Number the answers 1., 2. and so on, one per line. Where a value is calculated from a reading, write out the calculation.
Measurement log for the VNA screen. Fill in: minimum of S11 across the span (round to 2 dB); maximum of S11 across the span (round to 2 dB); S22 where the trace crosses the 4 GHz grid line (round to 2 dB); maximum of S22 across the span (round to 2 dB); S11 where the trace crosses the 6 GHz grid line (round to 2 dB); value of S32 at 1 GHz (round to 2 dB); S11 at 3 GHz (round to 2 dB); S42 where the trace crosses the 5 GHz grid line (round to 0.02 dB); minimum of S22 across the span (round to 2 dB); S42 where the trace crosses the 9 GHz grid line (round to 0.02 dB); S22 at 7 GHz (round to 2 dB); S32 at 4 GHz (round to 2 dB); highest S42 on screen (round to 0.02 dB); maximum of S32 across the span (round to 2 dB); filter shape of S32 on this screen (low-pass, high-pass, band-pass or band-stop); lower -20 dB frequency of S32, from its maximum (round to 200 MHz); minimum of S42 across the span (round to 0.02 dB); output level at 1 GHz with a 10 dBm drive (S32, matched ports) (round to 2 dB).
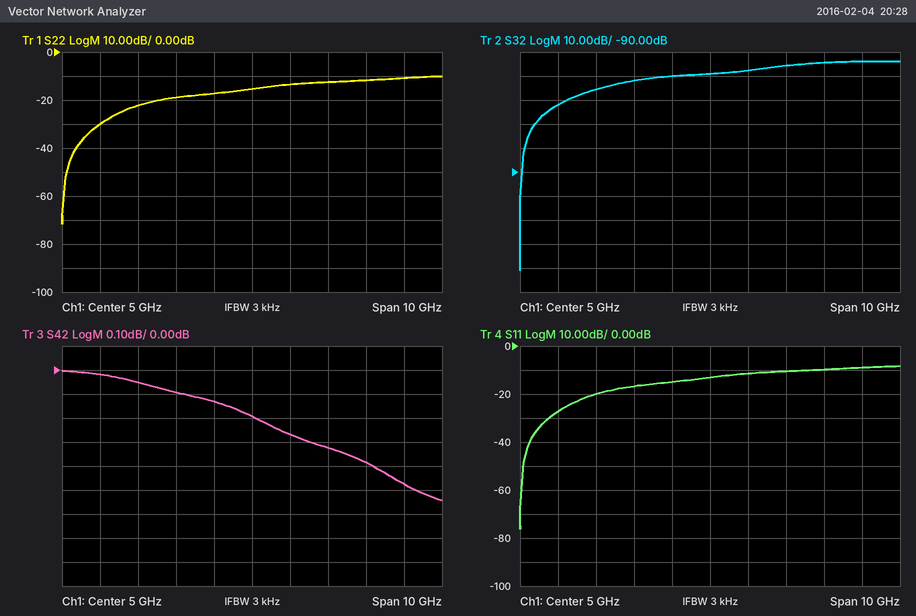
1. -76 dB
2. -8 dB
3. -18 dB
4. -10 dB
5. -12 dB
6. -62 dB
7. -16 dB
8. -0.20 dB
9. -72 dB
10. -0.48 dB
11. -12 dB
12. -50 dB
13. 0.00 dB
14. -44 dB
15. high-pass
16. 800 MHz
17. -0.54 dB
18. 10 dBm + (-62 dB) = -52 dBm
